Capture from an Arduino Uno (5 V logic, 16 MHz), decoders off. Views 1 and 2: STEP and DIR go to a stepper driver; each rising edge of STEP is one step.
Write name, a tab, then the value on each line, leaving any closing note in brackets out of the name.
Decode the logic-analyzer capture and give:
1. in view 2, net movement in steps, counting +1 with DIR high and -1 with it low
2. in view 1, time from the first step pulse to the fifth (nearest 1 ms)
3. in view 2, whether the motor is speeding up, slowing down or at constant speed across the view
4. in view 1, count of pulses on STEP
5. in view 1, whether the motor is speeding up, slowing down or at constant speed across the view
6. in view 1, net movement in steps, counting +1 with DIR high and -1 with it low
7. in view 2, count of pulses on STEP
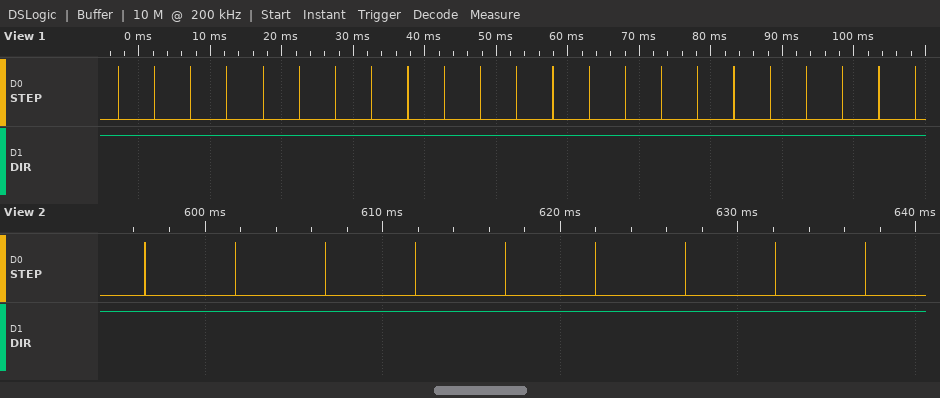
in view 2, net movement in steps, counting +1 with DIR high and -1 with it low	+9
in view 1, time from the first step pulse to the fifth	20 ms
in view 2, whether the motor is speeding up, slowing down or at constant speed across the view	constant speed
in view 1, count of pulses on STEP	23
in view 1, whether the motor is speeding up, slowing down or at constant speed across the view	constant speed
in view 1, net movement in steps, counting +1 with DIR high and -1 with it low	+23
in view 2, count of pulses on STEP	9
